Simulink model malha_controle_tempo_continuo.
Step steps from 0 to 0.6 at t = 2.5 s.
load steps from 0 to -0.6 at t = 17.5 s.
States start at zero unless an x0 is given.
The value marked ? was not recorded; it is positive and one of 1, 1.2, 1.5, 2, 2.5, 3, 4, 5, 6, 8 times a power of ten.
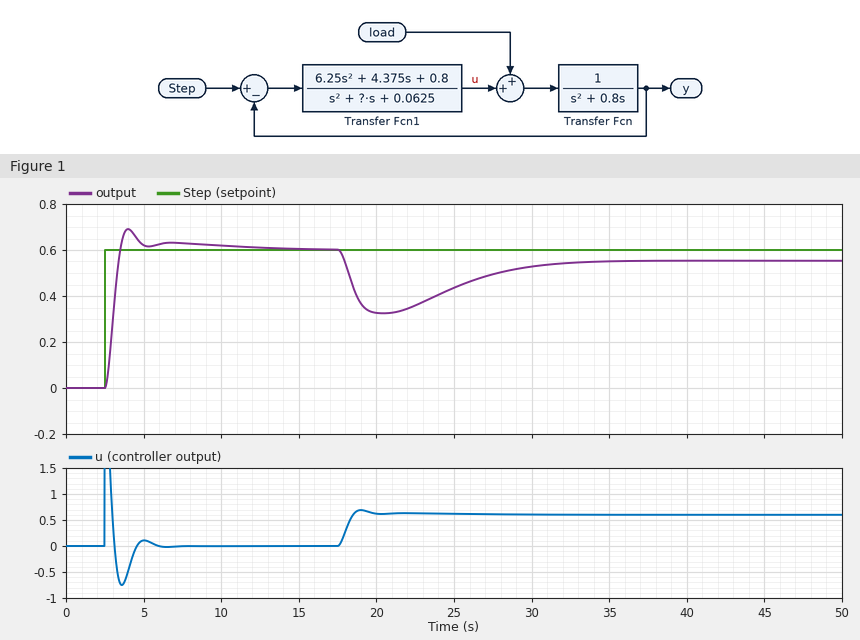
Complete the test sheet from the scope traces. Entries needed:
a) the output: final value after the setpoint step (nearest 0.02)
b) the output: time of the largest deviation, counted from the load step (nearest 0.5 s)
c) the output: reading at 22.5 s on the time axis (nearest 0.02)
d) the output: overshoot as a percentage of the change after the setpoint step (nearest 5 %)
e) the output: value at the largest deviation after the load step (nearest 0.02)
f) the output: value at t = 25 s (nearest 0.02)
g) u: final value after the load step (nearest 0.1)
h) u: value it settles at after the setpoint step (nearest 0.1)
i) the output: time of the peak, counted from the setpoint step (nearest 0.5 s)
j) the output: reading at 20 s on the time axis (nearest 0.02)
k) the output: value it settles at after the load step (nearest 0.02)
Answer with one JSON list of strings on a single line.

["0.60", "3.0 s", "0.36", "15 %", "0.32", "0.44", "0.6", "0.0", "1.5 s", "0.32", "0.56"]
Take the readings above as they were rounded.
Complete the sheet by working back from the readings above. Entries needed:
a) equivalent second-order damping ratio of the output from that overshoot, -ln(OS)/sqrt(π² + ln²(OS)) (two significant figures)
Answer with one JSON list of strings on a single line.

["0.52"]
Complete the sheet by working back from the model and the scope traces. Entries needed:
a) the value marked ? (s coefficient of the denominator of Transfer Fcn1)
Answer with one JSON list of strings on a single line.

["2.5"]
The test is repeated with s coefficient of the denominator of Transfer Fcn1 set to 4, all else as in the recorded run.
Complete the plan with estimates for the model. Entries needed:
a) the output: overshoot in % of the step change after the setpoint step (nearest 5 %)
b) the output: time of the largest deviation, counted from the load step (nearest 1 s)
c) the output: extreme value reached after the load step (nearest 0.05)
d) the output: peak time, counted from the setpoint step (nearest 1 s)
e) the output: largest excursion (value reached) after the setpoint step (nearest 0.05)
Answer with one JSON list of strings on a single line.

["10 %", "4 s", "0.15", "5 s", "0.65"]
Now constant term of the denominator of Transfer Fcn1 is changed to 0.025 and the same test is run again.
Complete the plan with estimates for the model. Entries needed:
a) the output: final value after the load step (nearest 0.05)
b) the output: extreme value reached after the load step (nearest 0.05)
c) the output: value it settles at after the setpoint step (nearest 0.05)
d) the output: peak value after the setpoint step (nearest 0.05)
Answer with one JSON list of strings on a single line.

["0.60", "0.35", "0.60", "0.70"]
